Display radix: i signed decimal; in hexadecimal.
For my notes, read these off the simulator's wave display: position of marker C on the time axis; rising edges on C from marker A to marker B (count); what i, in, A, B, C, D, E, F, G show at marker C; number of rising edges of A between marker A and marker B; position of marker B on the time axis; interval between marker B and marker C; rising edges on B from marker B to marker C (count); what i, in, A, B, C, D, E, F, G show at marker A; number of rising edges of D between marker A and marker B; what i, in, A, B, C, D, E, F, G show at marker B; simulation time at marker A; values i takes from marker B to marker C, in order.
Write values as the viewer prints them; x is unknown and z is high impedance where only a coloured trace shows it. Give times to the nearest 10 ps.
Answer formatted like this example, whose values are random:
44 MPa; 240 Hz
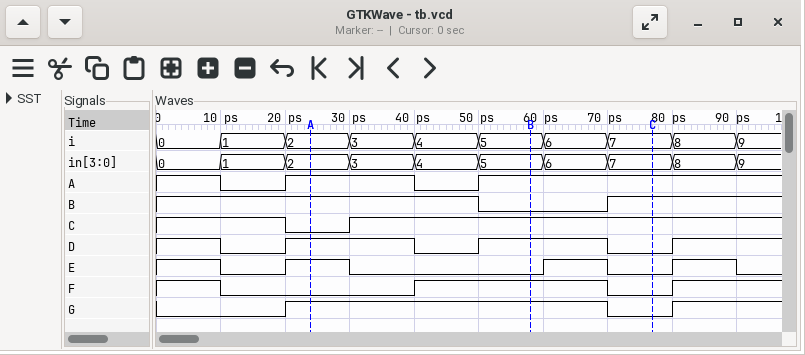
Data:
80 ps; 1; i=7, in=7, A=1, B=1, C=1, D=0, E=0, F=0, G=0; 1; 60 ps; 20 ps; 1; i=2, in=2, A=1, B=1, C=0, D=1, E=1, F=0, G=1; 1; i=5, in=5, A=1, B=0, C=1, D=1, E=0, F=1, G=1; 20 ps; 5, 6, 7
